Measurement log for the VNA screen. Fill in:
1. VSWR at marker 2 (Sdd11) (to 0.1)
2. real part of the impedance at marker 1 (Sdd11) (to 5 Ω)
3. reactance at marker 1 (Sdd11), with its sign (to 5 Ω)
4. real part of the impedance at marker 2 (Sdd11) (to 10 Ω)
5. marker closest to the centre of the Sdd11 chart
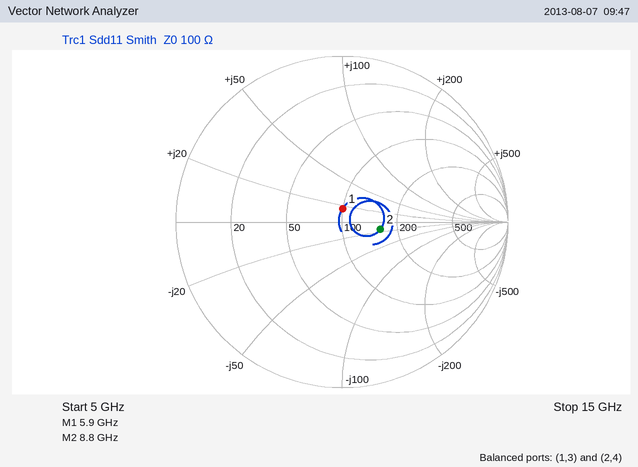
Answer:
1.6
100 Ω
+15 Ω
160 Ω
marker 1
